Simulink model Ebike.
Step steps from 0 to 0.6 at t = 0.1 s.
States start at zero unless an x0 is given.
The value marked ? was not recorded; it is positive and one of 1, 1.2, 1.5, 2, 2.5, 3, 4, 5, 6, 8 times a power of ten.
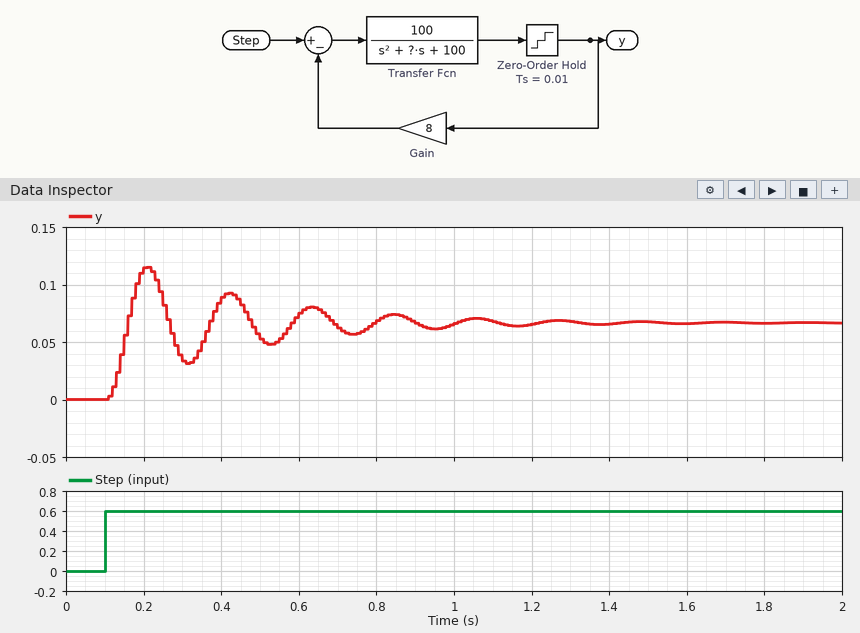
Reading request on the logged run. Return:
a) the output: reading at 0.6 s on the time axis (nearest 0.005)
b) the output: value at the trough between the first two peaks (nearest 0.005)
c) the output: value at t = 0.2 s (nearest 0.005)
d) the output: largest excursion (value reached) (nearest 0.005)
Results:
0.075
0.030
0.115
0.115
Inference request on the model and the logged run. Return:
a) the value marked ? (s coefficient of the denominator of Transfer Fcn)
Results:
10
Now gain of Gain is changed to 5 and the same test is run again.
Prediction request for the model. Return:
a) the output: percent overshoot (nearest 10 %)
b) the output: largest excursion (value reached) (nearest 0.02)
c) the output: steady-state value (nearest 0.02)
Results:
60 %
0.16
0.10
